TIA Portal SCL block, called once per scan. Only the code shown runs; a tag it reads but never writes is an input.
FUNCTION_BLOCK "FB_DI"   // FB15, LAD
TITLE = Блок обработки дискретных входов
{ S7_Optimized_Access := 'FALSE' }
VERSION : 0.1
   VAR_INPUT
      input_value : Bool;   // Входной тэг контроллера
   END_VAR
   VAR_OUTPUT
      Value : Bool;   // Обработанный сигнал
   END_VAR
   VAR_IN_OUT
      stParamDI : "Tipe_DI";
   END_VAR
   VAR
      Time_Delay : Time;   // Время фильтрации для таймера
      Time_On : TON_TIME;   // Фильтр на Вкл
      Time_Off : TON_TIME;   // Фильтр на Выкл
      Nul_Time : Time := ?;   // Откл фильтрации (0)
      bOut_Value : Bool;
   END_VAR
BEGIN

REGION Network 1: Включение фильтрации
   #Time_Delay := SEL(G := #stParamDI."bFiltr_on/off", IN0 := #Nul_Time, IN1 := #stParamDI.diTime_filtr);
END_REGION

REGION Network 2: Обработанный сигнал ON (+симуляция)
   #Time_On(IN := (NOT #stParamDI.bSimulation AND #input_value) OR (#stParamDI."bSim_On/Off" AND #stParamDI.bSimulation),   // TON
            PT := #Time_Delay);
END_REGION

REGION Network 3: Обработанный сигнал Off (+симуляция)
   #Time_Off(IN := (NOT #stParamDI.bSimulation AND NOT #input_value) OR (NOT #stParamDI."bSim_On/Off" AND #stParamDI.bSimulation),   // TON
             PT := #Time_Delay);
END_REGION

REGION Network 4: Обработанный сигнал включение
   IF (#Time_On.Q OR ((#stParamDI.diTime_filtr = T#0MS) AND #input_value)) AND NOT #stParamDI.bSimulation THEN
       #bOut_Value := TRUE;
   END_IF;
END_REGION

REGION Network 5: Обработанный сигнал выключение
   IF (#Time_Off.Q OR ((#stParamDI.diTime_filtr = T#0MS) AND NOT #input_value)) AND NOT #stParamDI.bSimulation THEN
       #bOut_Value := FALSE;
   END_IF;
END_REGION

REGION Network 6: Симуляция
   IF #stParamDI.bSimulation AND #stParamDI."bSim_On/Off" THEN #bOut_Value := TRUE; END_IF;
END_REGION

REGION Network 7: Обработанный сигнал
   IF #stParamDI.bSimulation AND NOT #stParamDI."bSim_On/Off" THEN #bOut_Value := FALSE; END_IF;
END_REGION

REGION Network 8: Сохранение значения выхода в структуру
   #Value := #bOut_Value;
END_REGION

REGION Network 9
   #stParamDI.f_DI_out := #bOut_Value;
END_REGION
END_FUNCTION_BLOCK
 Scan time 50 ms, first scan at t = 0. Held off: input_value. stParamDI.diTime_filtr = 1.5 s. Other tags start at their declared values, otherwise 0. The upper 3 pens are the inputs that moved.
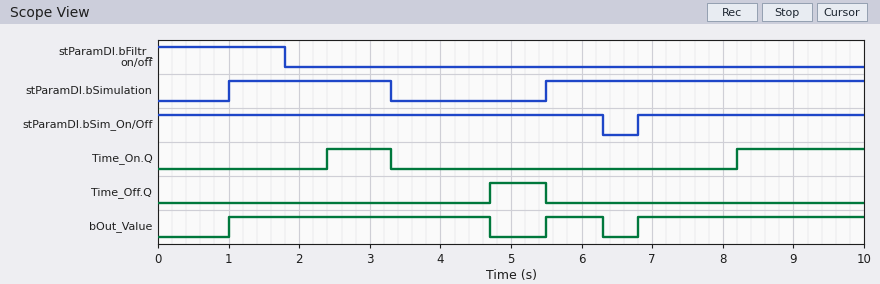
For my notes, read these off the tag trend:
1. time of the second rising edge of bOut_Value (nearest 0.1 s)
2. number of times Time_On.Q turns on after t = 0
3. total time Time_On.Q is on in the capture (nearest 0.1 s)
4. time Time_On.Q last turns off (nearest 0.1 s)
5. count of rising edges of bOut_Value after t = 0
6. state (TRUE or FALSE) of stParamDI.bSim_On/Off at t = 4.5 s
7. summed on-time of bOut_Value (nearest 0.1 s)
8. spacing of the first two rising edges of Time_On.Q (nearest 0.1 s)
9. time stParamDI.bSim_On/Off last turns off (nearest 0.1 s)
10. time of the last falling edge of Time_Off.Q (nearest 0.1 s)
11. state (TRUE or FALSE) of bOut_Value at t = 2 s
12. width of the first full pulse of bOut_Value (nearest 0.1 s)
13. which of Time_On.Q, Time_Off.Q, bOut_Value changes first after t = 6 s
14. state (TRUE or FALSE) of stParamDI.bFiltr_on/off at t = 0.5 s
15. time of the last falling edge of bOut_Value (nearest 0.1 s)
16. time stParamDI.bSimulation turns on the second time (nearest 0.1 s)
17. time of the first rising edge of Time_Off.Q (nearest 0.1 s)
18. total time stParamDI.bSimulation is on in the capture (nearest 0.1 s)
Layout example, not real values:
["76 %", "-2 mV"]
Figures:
["5.5 s", "2", "2.7 s", "3.3 s", "3", "TRUE", "7.7 s", "5.8 s", "6.3 s", "5.5 s", "TRUE", "3.7 s", "bOut_Value", "TRUE", "6.3 s", "5.5 s", "4.7 s", "6.8 s"]
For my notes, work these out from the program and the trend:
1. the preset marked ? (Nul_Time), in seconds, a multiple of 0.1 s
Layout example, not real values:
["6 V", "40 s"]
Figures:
["1.4 s"]
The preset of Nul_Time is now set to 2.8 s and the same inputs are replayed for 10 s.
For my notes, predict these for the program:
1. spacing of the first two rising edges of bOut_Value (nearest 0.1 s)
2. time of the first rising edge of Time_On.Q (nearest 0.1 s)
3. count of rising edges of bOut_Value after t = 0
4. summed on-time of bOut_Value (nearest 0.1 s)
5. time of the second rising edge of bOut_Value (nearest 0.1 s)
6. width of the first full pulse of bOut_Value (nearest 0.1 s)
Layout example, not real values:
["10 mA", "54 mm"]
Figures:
["5.8 s", "9.6 s", "2", "8.5 s", "6.8 s", "5.3 s"]
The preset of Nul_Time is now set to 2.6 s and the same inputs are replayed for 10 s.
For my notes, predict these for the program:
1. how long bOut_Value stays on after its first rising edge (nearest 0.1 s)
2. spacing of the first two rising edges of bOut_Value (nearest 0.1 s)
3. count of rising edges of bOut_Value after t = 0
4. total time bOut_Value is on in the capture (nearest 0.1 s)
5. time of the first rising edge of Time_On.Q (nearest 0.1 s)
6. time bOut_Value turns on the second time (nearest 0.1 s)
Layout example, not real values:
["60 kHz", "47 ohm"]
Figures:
["5.3 s", "5.8 s", "2", "8.5 s", "9.4 s", "6.8 s"]
